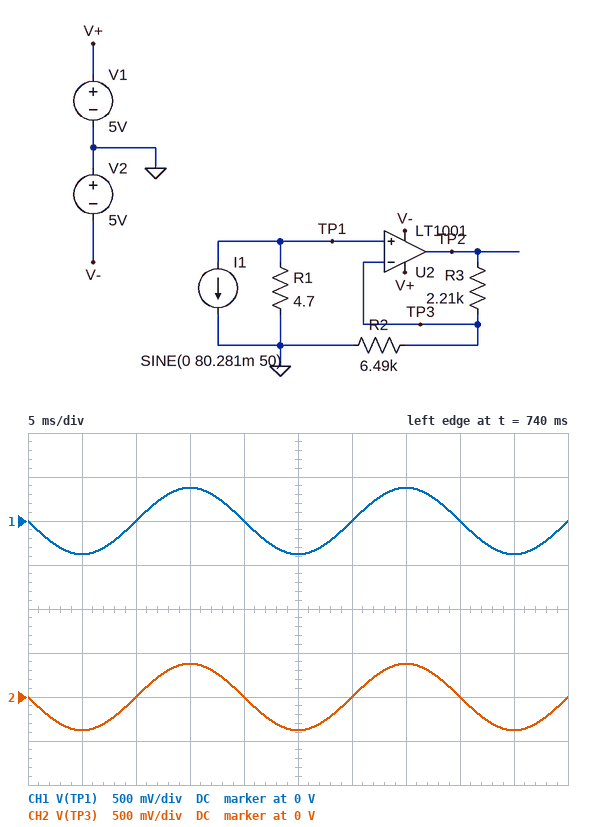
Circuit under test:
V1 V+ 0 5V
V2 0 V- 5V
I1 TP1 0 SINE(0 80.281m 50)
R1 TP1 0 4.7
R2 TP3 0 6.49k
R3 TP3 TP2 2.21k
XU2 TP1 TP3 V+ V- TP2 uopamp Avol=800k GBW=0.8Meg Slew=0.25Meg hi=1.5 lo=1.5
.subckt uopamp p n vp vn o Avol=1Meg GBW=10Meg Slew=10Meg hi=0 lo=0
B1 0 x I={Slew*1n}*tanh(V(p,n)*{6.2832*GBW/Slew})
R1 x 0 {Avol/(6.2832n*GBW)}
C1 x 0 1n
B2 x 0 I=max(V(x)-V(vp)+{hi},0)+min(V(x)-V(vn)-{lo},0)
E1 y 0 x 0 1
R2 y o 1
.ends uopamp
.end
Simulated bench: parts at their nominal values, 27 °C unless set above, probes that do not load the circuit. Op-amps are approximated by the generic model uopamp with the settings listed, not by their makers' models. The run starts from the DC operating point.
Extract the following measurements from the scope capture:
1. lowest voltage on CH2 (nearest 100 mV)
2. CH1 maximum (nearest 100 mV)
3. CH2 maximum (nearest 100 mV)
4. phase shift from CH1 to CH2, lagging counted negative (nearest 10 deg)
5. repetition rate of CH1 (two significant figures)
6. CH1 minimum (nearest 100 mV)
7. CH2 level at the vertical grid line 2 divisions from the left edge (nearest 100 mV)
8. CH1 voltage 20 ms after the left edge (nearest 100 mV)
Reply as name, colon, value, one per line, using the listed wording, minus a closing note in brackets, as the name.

lowest voltage on CH2: -400 mV
CH1 maximum: 400 mV
CH2 maximum: 400 mV
phase shift from CH1 to CH2, lagging counted negative: 0 deg
repetition rate of CH1: 50 Hz
CH1 minimum: -400 mV
CH2 level at the vertical grid line 2 divisions from the left edge: 0 V
CH1 voltage 20 ms after the left edge: 0 V
